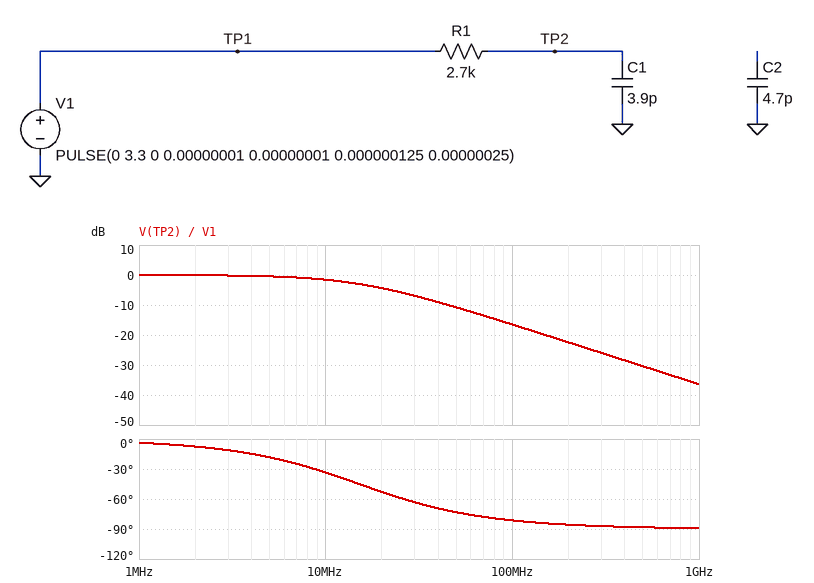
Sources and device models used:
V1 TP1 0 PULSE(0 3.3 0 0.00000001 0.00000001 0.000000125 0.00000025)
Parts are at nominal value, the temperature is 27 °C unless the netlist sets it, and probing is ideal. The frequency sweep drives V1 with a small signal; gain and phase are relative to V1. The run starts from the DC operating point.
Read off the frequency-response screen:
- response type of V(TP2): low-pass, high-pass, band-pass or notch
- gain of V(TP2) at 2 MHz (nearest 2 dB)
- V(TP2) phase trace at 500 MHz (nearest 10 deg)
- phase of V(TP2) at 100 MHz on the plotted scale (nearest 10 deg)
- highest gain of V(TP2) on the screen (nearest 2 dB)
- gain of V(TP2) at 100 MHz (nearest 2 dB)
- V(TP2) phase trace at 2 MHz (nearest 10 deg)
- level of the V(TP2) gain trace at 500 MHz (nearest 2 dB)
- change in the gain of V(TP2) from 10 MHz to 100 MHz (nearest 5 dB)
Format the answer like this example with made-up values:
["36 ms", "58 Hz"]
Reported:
["low-pass", "0 dB", "-90 deg", "-80 deg", "0 dB", "-16 dB", "-10 deg", "-30 dB", "-15 dB"]
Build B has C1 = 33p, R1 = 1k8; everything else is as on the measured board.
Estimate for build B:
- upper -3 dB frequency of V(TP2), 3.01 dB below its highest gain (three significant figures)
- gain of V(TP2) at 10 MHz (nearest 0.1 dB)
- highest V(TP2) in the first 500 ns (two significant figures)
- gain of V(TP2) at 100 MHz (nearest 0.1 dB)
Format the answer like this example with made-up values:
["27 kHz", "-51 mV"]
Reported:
["2.68 MHz", "-11.7 dB", "3.0 V", "-31.4 dB"]
